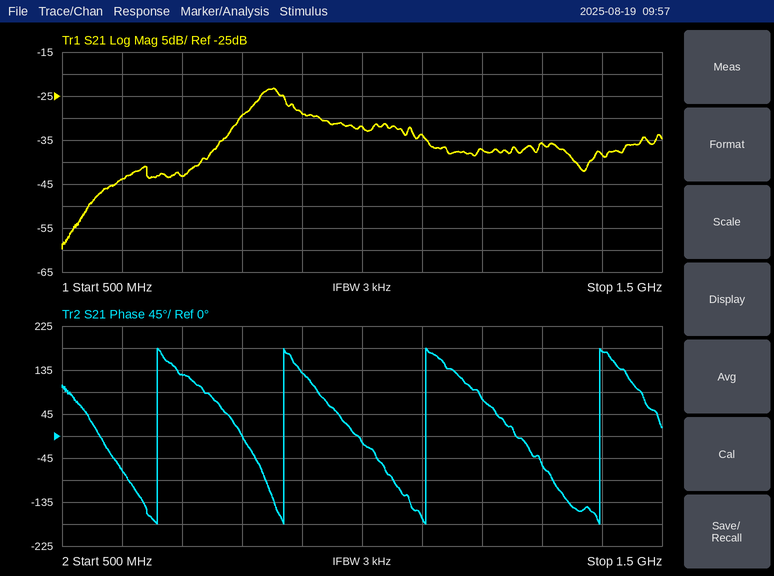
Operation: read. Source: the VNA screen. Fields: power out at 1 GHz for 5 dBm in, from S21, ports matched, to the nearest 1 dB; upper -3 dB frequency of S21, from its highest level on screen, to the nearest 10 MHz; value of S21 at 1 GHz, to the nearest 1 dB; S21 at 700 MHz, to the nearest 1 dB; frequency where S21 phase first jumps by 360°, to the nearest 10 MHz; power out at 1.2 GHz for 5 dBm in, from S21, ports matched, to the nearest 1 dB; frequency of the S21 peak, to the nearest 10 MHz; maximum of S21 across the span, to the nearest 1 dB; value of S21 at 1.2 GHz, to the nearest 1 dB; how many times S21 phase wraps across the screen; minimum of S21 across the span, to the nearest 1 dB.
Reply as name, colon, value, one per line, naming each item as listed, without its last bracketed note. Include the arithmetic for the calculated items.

power out at 1 GHz for 5 dBm in, from S21, ports matched, to the nearest 1 dB: 5 dBm + (-32 dB) = -27 dBm
upper -3 dB frequency of S21, from its highest level on screen, to the nearest 10 MHz: 870 MHz
value of S21 at 1 GHz, to the nearest 1 dB: -32 dB
S21 at 700 MHz, to the nearest 1 dB: -43 dB
frequency where S21 phase first jumps by 360°, to the nearest 10 MHz: 660 MHz
power out at 1.2 GHz for 5 dBm in, from S21, ports matched, to the nearest 1 dB: 5 dBm + (-37 dB) = -32 dBm
frequency of the S21 peak, to the nearest 10 MHz: 850 MHz
maximum of S21 across the span, to the nearest 1 dB: -23 dB
value of S21 at 1.2 GHz, to the nearest 1 dB: -37 dB
how many times S21 phase wraps across the screen: 4
minimum of S21 across the span, to the nearest 1 dB: -60 dB
